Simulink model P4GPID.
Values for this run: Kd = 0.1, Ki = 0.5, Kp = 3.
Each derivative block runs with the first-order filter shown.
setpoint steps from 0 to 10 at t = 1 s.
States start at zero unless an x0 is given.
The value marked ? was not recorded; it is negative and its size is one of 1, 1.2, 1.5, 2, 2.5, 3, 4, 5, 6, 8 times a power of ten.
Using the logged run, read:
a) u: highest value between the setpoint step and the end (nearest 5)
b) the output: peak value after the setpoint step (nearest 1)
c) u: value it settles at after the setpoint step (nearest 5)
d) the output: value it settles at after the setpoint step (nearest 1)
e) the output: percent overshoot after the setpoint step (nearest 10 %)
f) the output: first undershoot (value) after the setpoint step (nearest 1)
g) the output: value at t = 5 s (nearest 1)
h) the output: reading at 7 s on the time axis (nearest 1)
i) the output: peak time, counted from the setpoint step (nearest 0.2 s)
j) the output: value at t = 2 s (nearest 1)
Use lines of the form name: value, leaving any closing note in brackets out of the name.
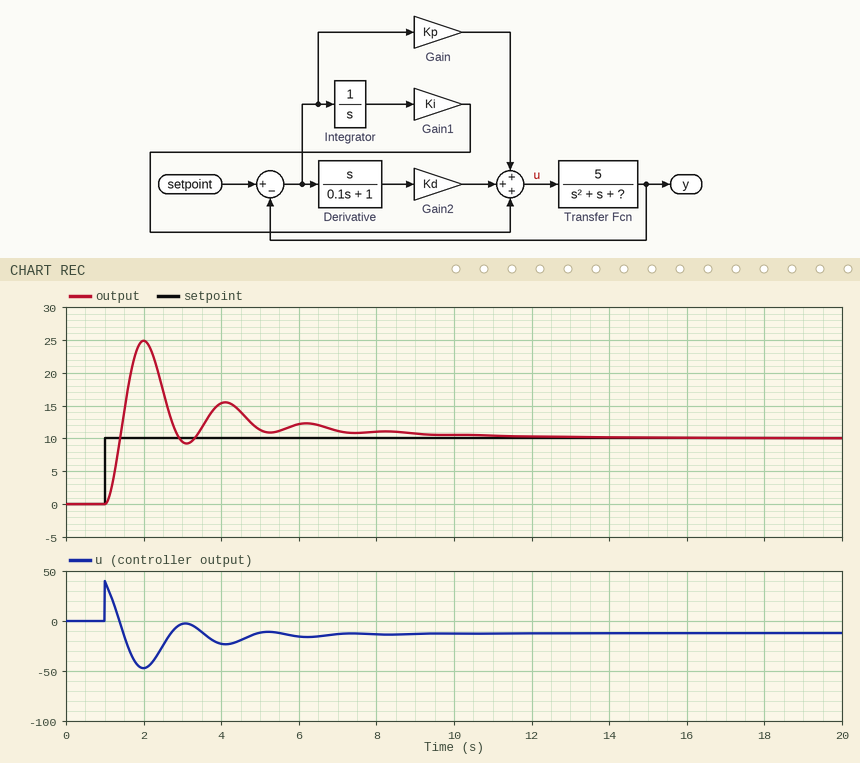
u: highest value between the setpoint step and the end: 40
the output: peak value after the setpoint step: 25
u: value it settles at after the setpoint step: -10
the output: value it settles at after the setpoint step: 10
the output: percent overshoot after the setpoint step: 150 %
the output: first undershoot (value) after the setpoint step: 9
the output: value at t = 5 s: 11
the output: reading at 7 s on the time axis: 11
the output: peak time, counted from the setpoint step: 1.0 s
the output: value at t = 2 s: 25
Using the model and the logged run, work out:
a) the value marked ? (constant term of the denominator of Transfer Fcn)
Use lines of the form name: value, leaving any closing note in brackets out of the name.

the value marked ?: -6
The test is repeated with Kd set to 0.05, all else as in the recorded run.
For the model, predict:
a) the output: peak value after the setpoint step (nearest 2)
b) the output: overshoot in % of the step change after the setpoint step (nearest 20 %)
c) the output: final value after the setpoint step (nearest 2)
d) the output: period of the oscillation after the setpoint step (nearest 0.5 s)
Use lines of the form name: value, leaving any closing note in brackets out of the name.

the output: peak value after the setpoint step: 26
the output: overshoot in % of the step change after the setpoint step: 160 %
the output: final value after the setpoint step: 10
the output: period of the oscillation after the setpoint step: 2.0 s
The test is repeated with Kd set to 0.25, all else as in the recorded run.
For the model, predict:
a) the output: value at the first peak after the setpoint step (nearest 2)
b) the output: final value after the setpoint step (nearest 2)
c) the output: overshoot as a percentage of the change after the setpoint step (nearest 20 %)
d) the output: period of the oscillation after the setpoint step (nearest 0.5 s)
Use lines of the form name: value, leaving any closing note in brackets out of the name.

the output: value at the first peak after the setpoint step: 22
the output: final value after the setpoint step: 10
the output: overshoot as a percentage of the change after the setpoint step: 120 %
the output: period of the oscillation after the setpoint step: 2.0 s
